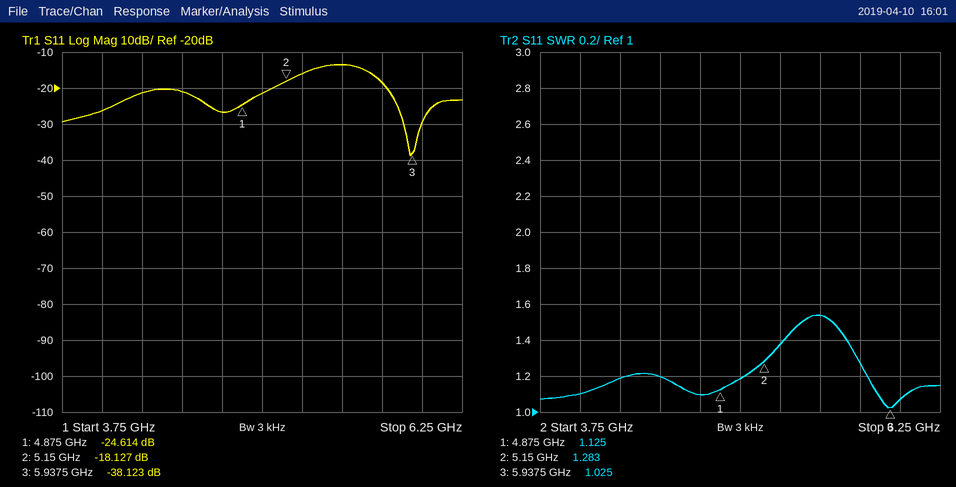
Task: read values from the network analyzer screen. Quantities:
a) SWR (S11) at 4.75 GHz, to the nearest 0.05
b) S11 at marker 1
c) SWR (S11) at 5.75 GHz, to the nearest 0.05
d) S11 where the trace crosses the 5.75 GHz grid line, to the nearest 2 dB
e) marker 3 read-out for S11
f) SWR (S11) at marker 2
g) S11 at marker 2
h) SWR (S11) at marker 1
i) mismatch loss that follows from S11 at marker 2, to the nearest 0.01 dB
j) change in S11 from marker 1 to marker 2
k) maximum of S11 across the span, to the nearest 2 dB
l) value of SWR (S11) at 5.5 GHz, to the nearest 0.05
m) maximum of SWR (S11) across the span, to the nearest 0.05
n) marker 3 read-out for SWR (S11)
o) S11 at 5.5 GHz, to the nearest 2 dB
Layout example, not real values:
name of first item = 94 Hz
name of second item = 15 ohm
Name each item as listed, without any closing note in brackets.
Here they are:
SWR (S11) at 4.75 GHz, to the nearest 0.05 = 1.10
S11 at marker 1 = -24.614 dB
SWR (S11) at 5.75 GHz, to the nearest 0.05 = 1.25
S11 where the trace crosses the 5.75 GHz grid line, to the nearest 2 dB = -18 dB
marker 3 read-out for S11 = -38.123 dB
SWR (S11) at marker 2 = 1.283
S11 at marker 2 = -18.127 dB
SWR (S11) at marker 1 = 1.125
mismatch loss that follows from S11 at marker 2, to the nearest 0.01 dB = 0.07 dB
change in S11 from marker 1 to marker 2 = 6.487 dB
maximum of S11 across the span, to the nearest 2 dB = -14 dB
value of SWR (S11) at 5.5 GHz, to the nearest 0.05 = 1.55
maximum of SWR (S11) across the span, to the nearest 0.05 = 1.55
marker 3 read-out for SWR = 1.025
S11 at 5.5 GHz, to the nearest 2 dB = -14 dB
